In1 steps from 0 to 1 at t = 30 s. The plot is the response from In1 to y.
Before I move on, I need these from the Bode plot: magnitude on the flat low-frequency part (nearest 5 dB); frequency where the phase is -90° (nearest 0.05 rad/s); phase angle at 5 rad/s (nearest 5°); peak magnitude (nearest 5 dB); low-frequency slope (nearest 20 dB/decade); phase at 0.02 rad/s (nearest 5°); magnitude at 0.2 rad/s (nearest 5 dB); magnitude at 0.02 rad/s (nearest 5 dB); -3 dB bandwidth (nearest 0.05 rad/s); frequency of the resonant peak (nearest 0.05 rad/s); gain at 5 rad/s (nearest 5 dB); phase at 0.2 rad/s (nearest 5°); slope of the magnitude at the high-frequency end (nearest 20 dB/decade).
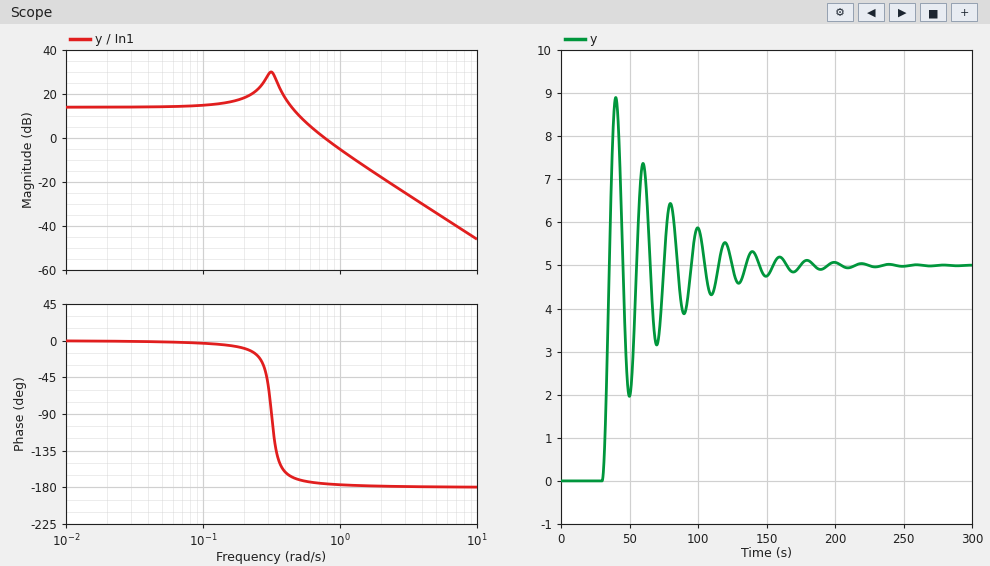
15 dB
0.30 rad/s
-180°
30 dB
0 dB/decade
0°
20 dB
15 dB
0.50 rad/s
0.30 rad/s
-35 dB
-10°
-40 dB/decade
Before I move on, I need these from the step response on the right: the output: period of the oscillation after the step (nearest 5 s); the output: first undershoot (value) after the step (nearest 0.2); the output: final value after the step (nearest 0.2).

20 s
2.0
5.0
